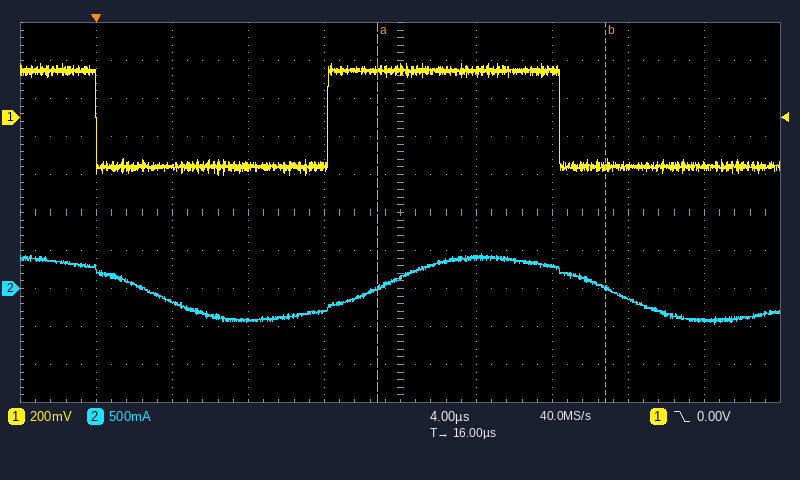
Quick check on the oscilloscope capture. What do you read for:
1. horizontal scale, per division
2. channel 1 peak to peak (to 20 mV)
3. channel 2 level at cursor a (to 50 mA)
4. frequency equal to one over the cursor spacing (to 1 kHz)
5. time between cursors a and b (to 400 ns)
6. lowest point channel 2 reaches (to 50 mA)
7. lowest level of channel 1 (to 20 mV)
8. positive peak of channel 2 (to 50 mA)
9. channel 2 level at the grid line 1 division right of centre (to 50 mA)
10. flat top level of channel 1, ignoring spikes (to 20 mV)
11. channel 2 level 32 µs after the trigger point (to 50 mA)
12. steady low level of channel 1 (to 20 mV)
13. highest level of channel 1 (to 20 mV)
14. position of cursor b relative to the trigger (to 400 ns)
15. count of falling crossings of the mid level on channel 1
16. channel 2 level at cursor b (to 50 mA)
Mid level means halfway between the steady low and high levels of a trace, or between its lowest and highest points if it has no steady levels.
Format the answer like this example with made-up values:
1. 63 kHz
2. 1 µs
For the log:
1. 4 µs
2. 580 mV
3. 0 mA
4. 83 kHz
5. 12.0 µs
6. -450 mA
7. -300 mV
8. 450 mA
9. 400 mA
10. 240 mV
11. -400 mA
12. -260 mV
13. 280 mV
14. +26.8 µs
15. 2
16. 0 mA
